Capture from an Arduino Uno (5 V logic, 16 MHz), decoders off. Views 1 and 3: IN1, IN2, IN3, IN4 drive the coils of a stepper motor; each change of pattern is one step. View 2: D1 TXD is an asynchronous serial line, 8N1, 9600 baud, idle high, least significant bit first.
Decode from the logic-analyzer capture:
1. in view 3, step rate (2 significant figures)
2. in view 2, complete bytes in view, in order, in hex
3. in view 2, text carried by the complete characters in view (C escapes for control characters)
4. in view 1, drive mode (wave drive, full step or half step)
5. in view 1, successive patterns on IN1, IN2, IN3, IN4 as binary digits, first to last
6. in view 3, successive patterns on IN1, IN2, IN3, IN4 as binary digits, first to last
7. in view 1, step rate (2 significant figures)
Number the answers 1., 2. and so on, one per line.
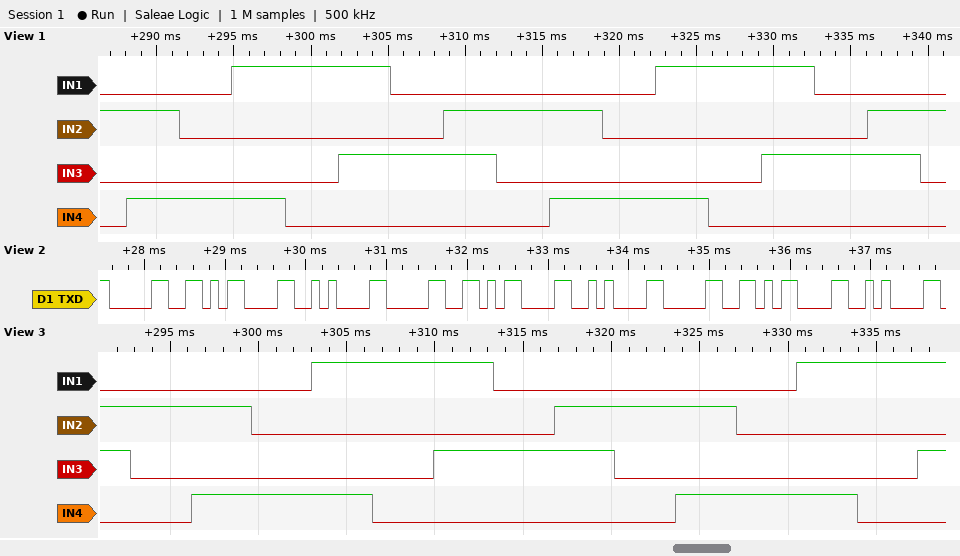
1. 290 steps/s
2. 30 0D 0A 30 0D 0A 30 0D 0A
3. "0\r\n0\r\n0\r\n"
4. half step
5. 0100 0101 0001 1001 1000 1010 0010 0110 0100 0101 0001 1001 1000 1010 0010 0110 0100
6. 0110 0100 0101 0001 1001 1000 1010 0010 0110 0100 0101 0001 1001 1000 1010
7. 290 steps/s
